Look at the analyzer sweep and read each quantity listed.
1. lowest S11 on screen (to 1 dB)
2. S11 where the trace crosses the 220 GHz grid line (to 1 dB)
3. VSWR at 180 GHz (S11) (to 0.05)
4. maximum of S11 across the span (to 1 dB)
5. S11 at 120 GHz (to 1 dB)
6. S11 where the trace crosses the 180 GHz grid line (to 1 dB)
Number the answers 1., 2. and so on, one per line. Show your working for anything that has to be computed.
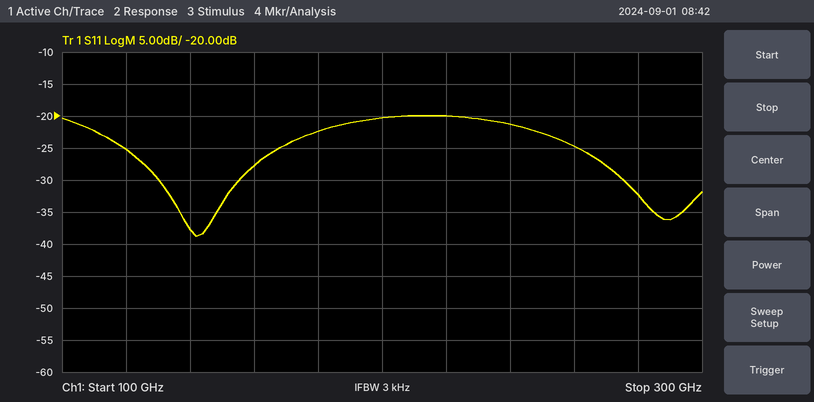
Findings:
1. -39 dB
2. -20 dB
3. |Γ| = 10^(-22/20) = 0.0794; VSWR = (1 + 0.0794)/(1 − 0.0794) ≈ 1.17, so 1.15 to the nearest 0.05
4. -20 dB
5. -25 dB
6. -22 dB
